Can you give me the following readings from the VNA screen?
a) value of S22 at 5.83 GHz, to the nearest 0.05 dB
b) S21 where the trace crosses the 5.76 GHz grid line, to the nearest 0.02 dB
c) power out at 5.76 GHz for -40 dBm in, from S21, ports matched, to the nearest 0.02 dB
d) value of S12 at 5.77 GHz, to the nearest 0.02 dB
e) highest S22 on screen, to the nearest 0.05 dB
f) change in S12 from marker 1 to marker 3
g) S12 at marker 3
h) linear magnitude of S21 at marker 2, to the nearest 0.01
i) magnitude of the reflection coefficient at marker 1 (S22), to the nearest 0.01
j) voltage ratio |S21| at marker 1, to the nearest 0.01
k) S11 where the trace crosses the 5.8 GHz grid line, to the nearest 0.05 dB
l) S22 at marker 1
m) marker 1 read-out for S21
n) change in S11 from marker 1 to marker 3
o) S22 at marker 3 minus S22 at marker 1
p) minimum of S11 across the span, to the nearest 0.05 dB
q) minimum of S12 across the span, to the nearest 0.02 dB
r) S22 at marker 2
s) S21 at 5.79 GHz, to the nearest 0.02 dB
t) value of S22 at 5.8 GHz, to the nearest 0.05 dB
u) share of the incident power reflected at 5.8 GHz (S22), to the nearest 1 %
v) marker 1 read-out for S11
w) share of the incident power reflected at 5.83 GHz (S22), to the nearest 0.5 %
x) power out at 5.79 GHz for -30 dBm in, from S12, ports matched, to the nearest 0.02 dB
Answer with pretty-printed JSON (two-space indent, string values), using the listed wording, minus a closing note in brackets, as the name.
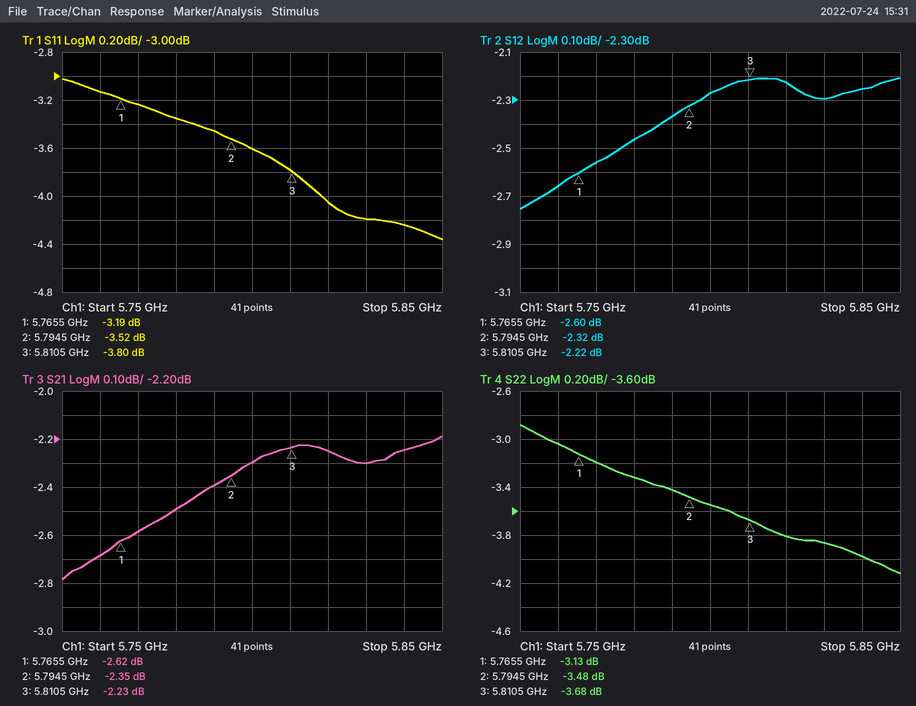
{
  "value of S22 at 5.83 GHz, to the nearest 0.05 dB": "-3.85 dB",
  "S21 where the trace crosses the 5.76 GHz grid line, to the nearest 0.02 dB": "-2.68 dB",
  "power out at 5.76 GHz for -40 dBm in, from S21, ports matched, to the nearest 0.02 dB": "-42.68 dBm",
  "value of S12 at 5.77 GHz, to the nearest 0.02 dB": "-2.56 dB",
  "highest S22 on screen, to the nearest 0.05 dB": "-2.90 dB",
  "change in S12 from marker 1 to marker 3": "0.38 dB",
  "S12 at marker 3": "-2.22 dB",
  "linear magnitude of S21 at marker 2, to the nearest 0.01": "0.76",
  "magnitude of the reflection coefficient at marker 1 (S22), to the nearest 0.01": "0.70",
  "voltage ratio |S21| at marker 1, to the nearest 0.01": "0.74",
  "S11 where the trace crosses the 5.8 GHz grid line, to the nearest 0.05 dB": "-3.60 dB",
  "S22 at marker 1": "-3.13 dB",
  "marker 1 read-out for S21": "-2.62 dB",
  "change in S11 from marker 1 to marker 3": "-0.61 dB",
  "S22 at marker 3 minus S22 at marker 1": "-0.55 dB",
  "minimum of S11 across the span, to the nearest 0.05 dB": "-4.35 dB",
  "minimum of S12 across the span, to the nearest 0.02 dB": "-2.76 dB",
  "S22 at marker 2": "-3.48 dB",
  "S21 at 5.79 GHz, to the nearest 0.02 dB": "-2.40 dB",
  "value of S22 at 5.8 GHz, to the nearest 0.05 dB": "-3.55 dB",
  "share of the incident power reflected at 5.8 GHz (S22), to the nearest 1 %": "44 %",
  "marker 1 read-out for S11": "-3.19 dB",
  "share of the incident power reflected at 5.83 GHz (S22), to the nearest 0.5 %": "41.0 %",
  "power out at 5.79 GHz for -30 dBm in, from S12, ports matched, to the nearest 0.02 dB": "-32.36 dBm"
}
